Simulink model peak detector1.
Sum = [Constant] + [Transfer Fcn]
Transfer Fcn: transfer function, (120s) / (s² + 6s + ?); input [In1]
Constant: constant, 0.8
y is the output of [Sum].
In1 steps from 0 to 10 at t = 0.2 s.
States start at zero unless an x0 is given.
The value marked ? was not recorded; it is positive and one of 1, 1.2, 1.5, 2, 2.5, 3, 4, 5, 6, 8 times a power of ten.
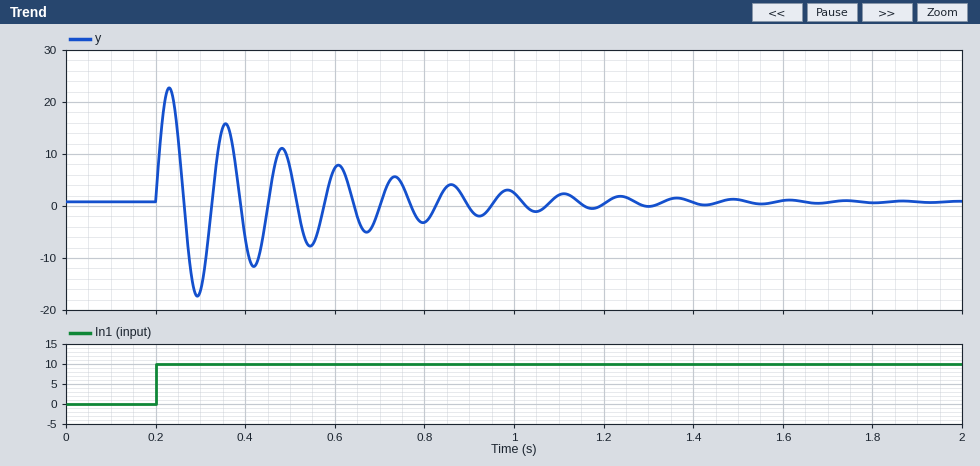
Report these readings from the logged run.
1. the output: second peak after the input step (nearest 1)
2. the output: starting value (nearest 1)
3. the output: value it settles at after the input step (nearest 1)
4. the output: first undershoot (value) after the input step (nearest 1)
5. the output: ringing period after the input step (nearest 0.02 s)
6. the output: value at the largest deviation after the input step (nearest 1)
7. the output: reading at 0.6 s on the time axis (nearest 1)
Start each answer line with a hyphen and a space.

- 16
- 1
- 1
- -17
- 0.12 s
- 23
- 7
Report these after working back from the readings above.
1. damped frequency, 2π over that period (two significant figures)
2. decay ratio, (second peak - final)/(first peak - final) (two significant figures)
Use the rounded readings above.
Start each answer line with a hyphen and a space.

- 52 rad/s
- 0.68
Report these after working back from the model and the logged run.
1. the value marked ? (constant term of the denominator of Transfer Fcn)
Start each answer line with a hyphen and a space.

- 2500
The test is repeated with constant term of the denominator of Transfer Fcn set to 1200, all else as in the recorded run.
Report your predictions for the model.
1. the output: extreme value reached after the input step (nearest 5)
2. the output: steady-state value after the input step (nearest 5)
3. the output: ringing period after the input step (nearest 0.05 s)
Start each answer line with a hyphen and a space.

- 30
- 0
- 0.20 s
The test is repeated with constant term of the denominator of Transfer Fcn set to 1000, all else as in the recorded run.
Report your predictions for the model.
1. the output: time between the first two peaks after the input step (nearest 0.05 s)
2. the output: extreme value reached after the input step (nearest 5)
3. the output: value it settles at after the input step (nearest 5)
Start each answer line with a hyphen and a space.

- 0.20 s
- 35
- 0
